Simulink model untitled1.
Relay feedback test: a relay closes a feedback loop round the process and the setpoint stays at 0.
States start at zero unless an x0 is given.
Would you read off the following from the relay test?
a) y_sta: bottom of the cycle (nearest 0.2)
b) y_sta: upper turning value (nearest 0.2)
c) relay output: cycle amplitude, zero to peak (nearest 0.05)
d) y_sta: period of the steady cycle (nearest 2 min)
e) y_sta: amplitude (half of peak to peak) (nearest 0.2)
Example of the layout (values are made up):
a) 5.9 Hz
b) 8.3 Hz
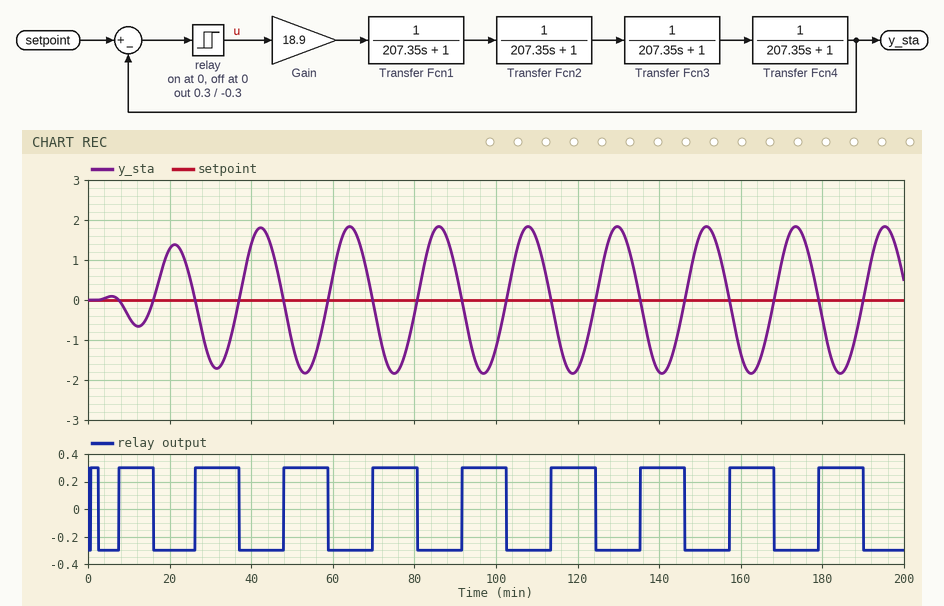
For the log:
a) -1.8
b) 1.8
c) 0.30
d) 22 min
e) 1.8
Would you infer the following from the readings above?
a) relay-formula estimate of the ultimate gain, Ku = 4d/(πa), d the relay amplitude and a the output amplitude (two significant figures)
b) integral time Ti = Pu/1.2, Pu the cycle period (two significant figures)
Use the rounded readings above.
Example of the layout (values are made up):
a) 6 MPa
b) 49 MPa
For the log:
a) 0.21
b) 18 min
